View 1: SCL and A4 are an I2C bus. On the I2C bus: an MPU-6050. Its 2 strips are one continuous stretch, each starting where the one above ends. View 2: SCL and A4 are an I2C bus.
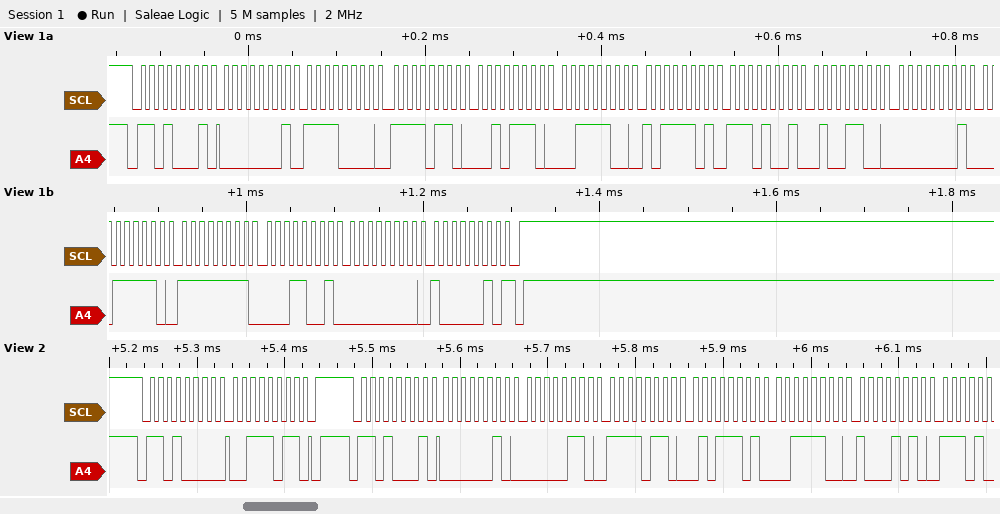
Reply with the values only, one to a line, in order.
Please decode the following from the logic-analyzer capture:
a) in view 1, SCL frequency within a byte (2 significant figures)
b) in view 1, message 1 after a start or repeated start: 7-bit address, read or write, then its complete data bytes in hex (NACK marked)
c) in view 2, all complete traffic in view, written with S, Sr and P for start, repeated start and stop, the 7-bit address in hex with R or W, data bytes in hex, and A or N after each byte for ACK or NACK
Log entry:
100 kHz
0x68 read: 01 F0 F6 2E 3C BD E9 4C 01 3E FF 19 00 82 NACK
S 68W A 3B A P S 68R A 02 A 06 A F6 A 5D A 3C A 8A A
